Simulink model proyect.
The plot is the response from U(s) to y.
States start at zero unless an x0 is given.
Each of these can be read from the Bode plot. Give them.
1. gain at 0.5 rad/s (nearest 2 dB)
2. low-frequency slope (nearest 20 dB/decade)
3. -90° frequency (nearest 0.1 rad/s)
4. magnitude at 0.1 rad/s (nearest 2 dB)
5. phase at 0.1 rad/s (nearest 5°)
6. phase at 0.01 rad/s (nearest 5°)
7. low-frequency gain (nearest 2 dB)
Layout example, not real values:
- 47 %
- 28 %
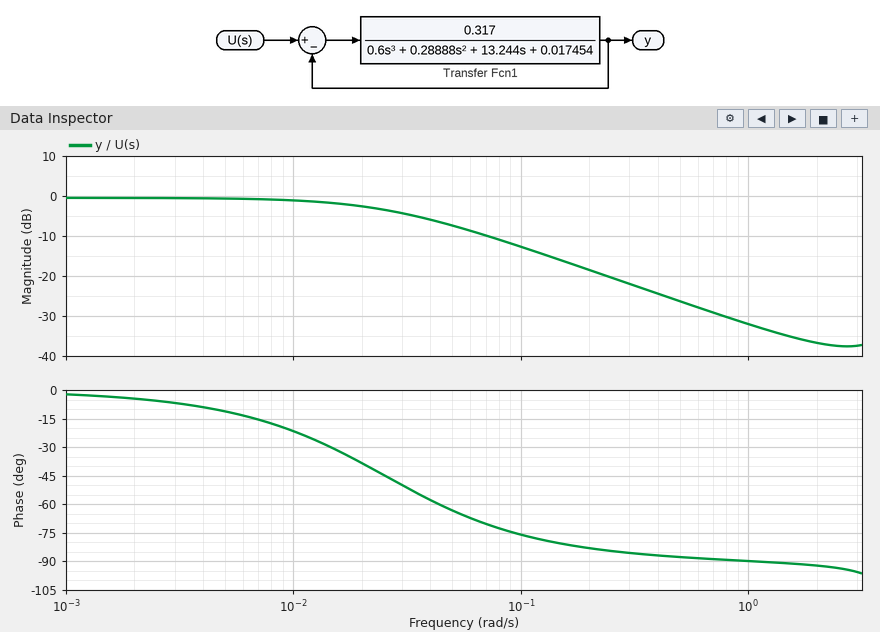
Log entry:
- -26 dB
- 0 dB/decade
- 1.1 rad/s
- -12 dB
- -75°
- -20°
- 0 dB
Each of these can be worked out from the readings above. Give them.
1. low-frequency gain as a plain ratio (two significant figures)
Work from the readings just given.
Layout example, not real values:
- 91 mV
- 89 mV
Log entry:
- 1.0
